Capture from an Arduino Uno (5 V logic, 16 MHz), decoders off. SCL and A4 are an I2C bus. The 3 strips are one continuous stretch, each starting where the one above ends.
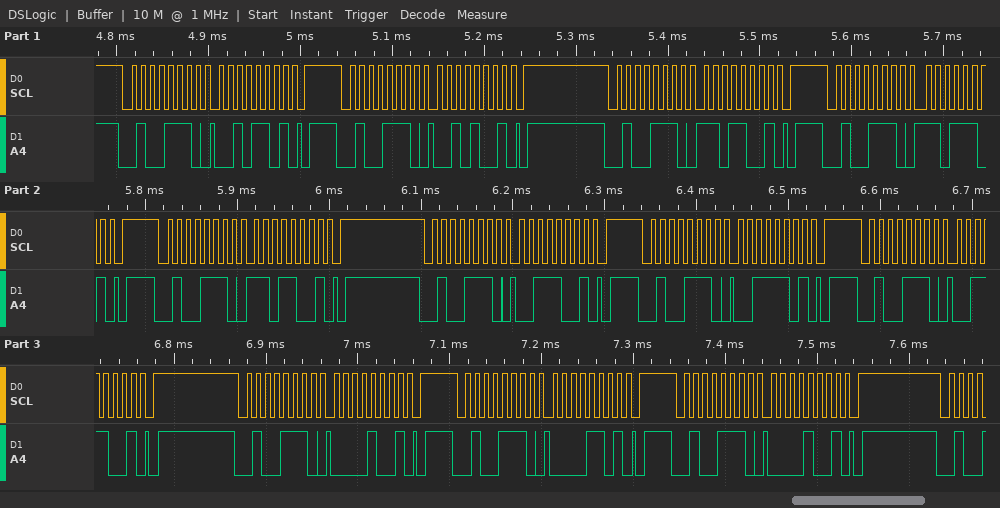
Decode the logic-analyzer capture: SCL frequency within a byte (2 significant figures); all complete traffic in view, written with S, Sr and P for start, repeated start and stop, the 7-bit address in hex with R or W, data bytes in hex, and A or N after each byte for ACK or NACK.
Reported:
100 kHz
S 27W A 2D A P S 27W A 29 A P S 27W A D9 A P S 27W A DD A P S 27W A D9 A P S 27W A 39 A P S 27W A 3D A P S 27W A 39 A P S 27W A 09 A P S 27W A 0D A P S 27W A 09 A P
